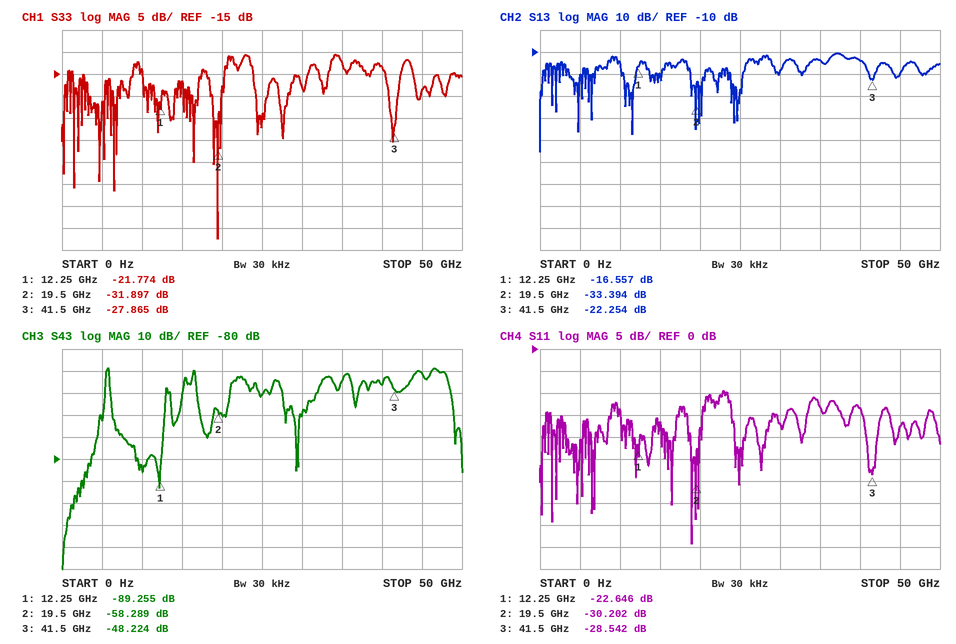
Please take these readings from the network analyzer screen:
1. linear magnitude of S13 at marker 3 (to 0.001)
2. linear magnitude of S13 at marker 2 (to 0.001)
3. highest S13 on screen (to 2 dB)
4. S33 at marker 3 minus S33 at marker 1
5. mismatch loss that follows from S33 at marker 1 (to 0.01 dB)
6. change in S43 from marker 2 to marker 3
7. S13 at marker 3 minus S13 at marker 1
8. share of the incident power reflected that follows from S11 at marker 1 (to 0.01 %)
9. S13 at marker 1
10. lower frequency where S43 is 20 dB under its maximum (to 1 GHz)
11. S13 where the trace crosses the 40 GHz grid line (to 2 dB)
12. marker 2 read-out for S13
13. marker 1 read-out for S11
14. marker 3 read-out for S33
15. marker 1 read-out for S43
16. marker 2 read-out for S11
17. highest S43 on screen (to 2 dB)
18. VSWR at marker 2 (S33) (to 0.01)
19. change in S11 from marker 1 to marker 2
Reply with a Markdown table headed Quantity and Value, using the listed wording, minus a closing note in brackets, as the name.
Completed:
| Quantity | Value |
|---|---|
| linear magnitude of S13 at marker 3 | 0.077 |
| linear magnitude of S13 at marker 2 | 0.021 |
| highest S13 on screen | -10 dB |
| S33 at marker 3 minus S33 at marker 1 | -6.091 dB |
| mismatch loss that follows from S33 at marker 1 | 0.03 dB |
| change in S43 from marker 2 to marker 3 | 10.065 dB |
| S13 at marker 3 minus S13 at marker 1 | -5.697 dB |
| share of the incident power reflected that follows from S11 at marker 1 | 0.54 % |
| S13 at marker 1 | -16.557 dB |
| lower frequency where S43 is 20 dB under its maximum | 5 GHz |
| S13 where the trace crosses the 40 GHz grid line | -14 dB |
| marker 2 read-out for S13 | -33.394 dB |
| marker 1 read-out for S11 | -22.646 dB |
| marker 3 read-out for S33 | -27.865 dB |
| marker 1 read-out for S43 | -89.255 dB |
| marker 2 read-out for S11 | -30.202 dB |
| highest S43 on screen | -38 dB |
| VSWR at marker 2 (S33) | 1.05 |
| change in S11 from marker 1 to marker 2 | -7.556 dB |
